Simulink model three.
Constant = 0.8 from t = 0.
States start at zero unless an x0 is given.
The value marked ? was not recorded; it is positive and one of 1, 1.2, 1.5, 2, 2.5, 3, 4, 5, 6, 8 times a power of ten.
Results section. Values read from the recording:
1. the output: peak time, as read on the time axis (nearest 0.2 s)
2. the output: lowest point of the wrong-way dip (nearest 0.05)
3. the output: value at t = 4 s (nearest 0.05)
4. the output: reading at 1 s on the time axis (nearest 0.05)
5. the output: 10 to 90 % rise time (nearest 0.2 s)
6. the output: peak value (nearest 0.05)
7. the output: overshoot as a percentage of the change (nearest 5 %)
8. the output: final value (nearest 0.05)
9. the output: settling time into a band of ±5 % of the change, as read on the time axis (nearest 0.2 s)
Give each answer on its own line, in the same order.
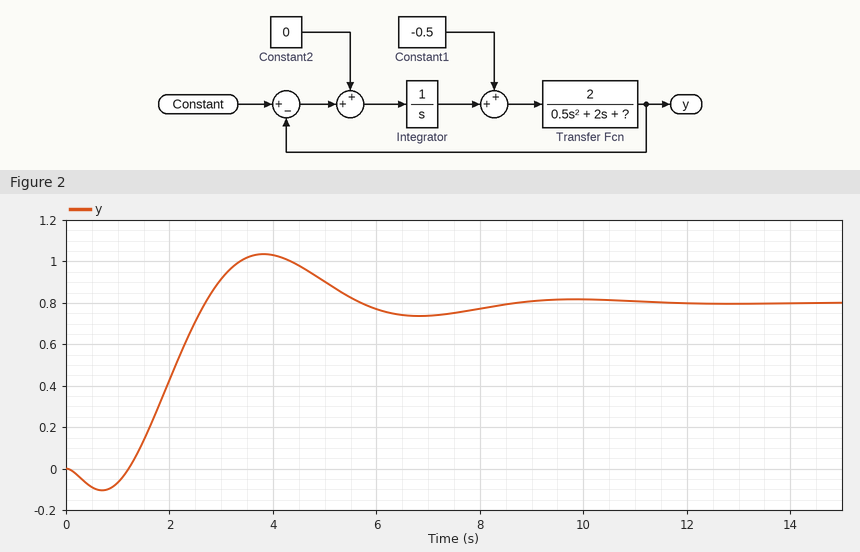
3.8 s
-0.10
1.05
-0.05
1.2 s
1.05
30 %
0.80
7.8 s
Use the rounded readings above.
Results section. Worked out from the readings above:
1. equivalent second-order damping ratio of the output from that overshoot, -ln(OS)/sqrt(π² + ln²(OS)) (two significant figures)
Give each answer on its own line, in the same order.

0.36
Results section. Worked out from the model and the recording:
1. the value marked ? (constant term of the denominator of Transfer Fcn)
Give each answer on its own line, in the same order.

2
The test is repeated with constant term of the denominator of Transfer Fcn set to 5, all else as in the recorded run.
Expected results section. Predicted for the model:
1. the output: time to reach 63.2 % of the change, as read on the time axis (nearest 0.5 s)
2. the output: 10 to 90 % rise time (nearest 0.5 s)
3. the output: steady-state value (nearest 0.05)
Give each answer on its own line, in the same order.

3.0 s
4.5 s
0.80
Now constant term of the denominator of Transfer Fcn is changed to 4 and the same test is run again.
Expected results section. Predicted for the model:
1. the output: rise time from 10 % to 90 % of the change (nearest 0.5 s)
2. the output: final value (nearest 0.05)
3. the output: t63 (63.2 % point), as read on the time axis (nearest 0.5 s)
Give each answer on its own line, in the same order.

3.0 s
0.80
2.5 s
